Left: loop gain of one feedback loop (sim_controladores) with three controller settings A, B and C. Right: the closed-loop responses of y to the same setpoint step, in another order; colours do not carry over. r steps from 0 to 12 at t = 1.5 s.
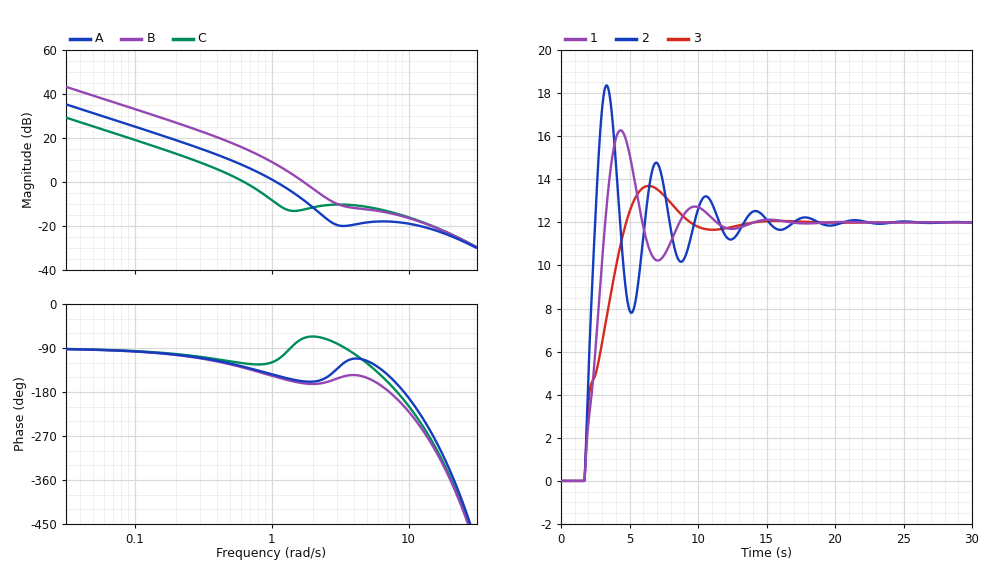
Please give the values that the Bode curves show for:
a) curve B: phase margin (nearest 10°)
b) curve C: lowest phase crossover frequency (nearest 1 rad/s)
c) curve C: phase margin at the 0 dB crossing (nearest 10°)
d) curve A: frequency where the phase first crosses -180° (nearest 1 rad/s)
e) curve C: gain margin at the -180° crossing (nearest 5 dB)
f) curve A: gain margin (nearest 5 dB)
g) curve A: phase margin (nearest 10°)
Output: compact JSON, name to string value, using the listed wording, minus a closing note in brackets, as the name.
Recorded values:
{"curve B: phase margin": "20°", "curve C: lowest phase crossover frequency": "8 rad/s", "curve C: phase margin at the 0 dB crossing": "60°", "curve A: frequency where the phase first crosses -180°": "9 rad/s", "curve C: gain margin at the -180° crossing": "15 dB", "curve A: gain margin": "20 dB", "curve A: phase margin": "30°"}
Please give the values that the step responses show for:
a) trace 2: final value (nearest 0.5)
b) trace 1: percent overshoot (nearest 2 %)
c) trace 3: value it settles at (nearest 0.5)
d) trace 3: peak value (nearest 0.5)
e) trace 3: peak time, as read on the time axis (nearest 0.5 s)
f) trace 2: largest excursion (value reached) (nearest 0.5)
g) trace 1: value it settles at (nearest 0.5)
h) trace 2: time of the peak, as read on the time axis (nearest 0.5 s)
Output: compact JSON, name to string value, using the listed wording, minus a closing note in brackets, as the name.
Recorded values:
{"trace 2: final value": "12.0", "trace 1: percent overshoot": "36 %", "trace 3: value it settles at": "12.0", "trace 3: peak value": "13.5", "trace 3: peak time, as read on the time axis": "6.5 s", "trace 2: largest excursion (value reached)": "18.5", "trace 1: value it settles at": "12.0", "trace 2: time of the peak, as read on the time axis": "3.5 s"}
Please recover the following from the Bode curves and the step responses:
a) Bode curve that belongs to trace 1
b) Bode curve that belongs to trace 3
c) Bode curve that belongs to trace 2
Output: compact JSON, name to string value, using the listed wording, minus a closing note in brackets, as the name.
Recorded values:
{"Bode curve that belongs to trace 1": "A", "Bode curve that belongs to trace 3": "C", "Bode curve that belongs to trace 2": "B"}
